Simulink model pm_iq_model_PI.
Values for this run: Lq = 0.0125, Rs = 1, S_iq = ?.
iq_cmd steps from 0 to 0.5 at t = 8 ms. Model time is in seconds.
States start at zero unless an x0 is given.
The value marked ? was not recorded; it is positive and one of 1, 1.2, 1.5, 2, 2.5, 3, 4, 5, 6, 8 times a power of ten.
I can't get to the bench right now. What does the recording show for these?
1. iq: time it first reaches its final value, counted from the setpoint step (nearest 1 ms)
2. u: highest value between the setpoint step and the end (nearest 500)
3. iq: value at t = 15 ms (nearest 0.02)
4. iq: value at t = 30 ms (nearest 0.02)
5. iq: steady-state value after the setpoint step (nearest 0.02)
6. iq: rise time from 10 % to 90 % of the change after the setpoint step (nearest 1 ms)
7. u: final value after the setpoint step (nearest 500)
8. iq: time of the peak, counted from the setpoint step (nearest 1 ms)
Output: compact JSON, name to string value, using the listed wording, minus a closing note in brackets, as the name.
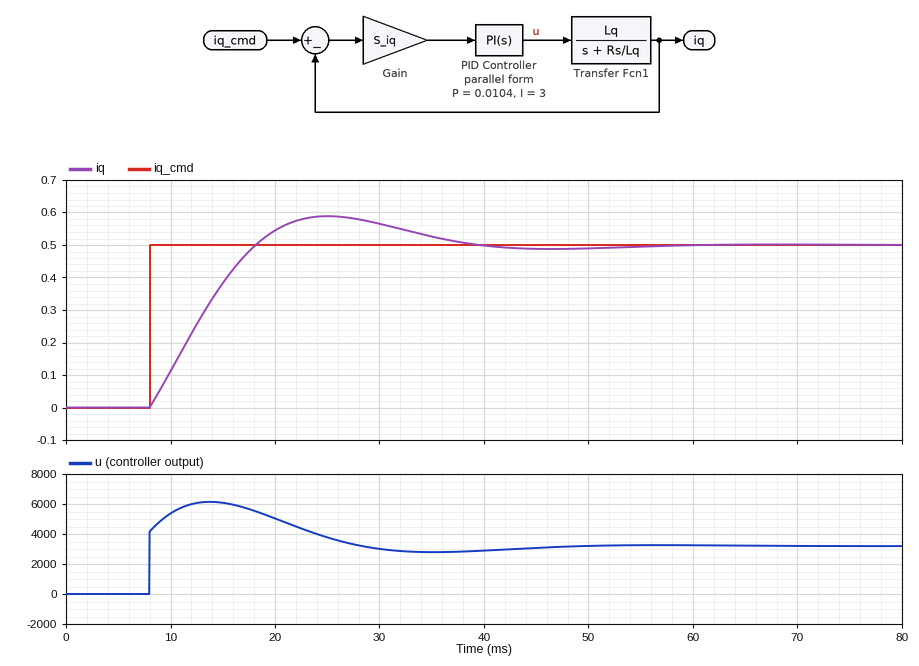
{"iq: time it first reaches its final value, counted from the setpoint step": "10 ms", "u: highest value between the setpoint step and the end": "6000", "iq: value at t = 15 ms": "0.38", "iq: value at t = 30 ms": "0.56", "iq: steady-state value after the setpoint step": "0.50", "iq: rise time from 10 % to 90 % of the change after the setpoint step": "8 ms", "u: final value after the setpoint step": "3000", "iq: time of the peak, counted from the setpoint step": "17 ms"}
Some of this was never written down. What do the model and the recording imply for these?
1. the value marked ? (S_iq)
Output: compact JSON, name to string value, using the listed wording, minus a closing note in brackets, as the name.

{"the value marked ?": "800000"}
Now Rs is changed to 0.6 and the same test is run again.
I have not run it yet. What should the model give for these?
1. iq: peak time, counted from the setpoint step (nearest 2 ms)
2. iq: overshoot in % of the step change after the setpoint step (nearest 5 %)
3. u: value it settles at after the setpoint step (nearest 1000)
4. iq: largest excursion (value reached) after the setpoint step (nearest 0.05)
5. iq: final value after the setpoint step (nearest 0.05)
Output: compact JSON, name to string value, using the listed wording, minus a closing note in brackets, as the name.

{"iq: peak time, counted from the setpoint step": "16 ms", "iq: overshoot in % of the step change after the setpoint step": "25 %", "u: value it settles at after the setpoint step": "2000", "iq: largest excursion (value reached) after the setpoint step": "0.65", "iq: final value after the setpoint step": "0.50"}
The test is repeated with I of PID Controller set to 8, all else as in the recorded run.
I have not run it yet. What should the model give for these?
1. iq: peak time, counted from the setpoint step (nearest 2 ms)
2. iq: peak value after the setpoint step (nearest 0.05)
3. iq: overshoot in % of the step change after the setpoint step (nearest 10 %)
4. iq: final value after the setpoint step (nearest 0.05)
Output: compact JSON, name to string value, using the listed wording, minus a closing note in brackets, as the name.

{"iq: peak time, counted from the setpoint step": "10 ms", "iq: peak value after the setpoint step": "0.70", "iq: overshoot in % of the step change after the setpoint step": "40 %", "iq: final value after the setpoint step": "0.50"}
